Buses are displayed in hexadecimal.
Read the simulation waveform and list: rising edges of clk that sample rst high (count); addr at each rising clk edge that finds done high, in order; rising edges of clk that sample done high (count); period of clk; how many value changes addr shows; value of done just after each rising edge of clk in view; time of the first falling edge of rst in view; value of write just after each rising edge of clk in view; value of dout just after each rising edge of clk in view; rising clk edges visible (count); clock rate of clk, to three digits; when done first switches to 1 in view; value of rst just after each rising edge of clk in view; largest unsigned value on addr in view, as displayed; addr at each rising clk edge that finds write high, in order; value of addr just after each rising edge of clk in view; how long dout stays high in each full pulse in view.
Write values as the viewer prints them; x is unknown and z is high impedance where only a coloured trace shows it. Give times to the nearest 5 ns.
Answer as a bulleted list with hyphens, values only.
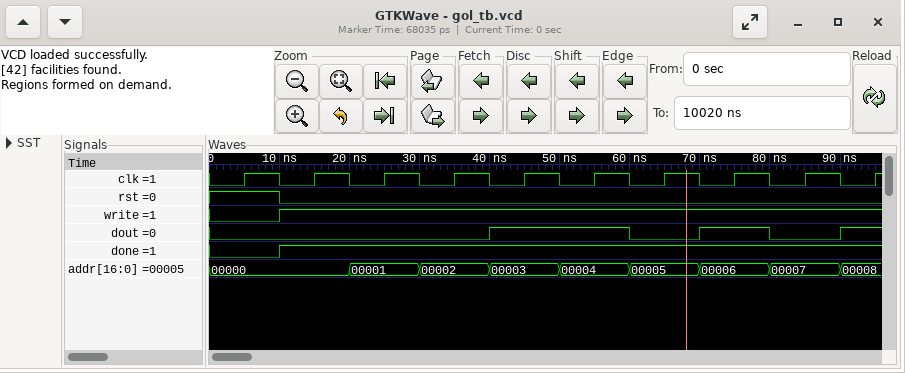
- 1
- 00000, 00001, 00002, 00003, 00004, 00005, 00006, 00007, 00008
- 9
- 10 ns
- 8
- 0 1 1 1 1 1 1 1 1 1
- 10 ns
- 0 1 1 1 1 1 1 1 1 1
- 0 0 0 0 1 1 0 1 0 1
- 10
- 100 MHz
- 10 ns
- 1 0 0 0 0 0 0 0 0 0
- 00008
- 00000, 00001, 00002, 00003, 00004, 00005, 00006, 00007, 00008
- 00000, 00000, 00001, 00002, 00003, 00004, 00005, 00006, 00007, 00008
- 20 ns, 10 ns
